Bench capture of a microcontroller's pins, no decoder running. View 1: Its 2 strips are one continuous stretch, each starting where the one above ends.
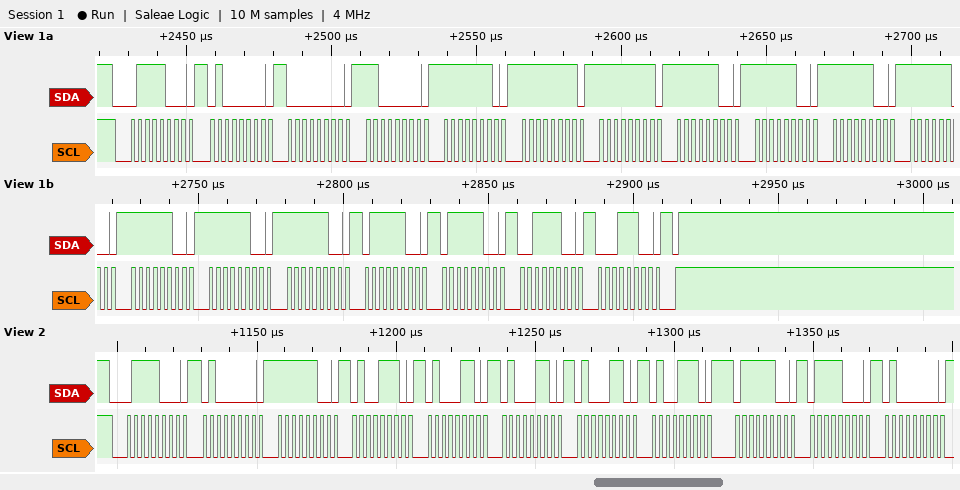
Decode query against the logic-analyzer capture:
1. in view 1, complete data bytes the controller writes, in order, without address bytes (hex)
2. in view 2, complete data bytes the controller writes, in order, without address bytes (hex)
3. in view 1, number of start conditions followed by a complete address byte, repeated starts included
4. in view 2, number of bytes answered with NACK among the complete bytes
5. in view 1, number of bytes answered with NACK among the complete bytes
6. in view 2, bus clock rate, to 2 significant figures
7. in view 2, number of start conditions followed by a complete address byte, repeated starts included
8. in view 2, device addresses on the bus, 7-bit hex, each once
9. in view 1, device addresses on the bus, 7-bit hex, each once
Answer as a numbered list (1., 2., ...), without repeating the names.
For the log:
1. 40 00 C0 FE FF FF FC FC FC FC FC FC FC 7C 7C 3C 1C
2. 40 FC 4E 46 46 46 4E 7C 78 40
3. 1
4. 0
5. 0
6. 400 kHz
7. 1
8. 0x3C
9. 0x3C
